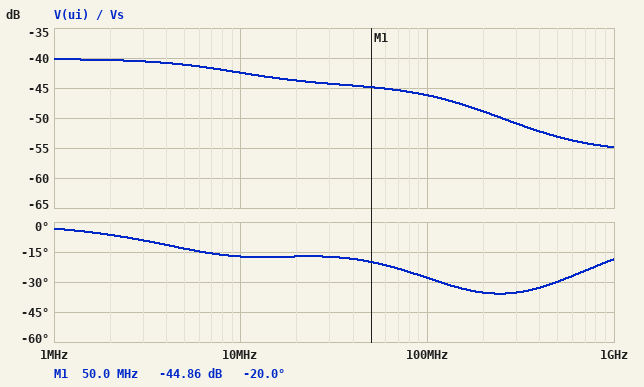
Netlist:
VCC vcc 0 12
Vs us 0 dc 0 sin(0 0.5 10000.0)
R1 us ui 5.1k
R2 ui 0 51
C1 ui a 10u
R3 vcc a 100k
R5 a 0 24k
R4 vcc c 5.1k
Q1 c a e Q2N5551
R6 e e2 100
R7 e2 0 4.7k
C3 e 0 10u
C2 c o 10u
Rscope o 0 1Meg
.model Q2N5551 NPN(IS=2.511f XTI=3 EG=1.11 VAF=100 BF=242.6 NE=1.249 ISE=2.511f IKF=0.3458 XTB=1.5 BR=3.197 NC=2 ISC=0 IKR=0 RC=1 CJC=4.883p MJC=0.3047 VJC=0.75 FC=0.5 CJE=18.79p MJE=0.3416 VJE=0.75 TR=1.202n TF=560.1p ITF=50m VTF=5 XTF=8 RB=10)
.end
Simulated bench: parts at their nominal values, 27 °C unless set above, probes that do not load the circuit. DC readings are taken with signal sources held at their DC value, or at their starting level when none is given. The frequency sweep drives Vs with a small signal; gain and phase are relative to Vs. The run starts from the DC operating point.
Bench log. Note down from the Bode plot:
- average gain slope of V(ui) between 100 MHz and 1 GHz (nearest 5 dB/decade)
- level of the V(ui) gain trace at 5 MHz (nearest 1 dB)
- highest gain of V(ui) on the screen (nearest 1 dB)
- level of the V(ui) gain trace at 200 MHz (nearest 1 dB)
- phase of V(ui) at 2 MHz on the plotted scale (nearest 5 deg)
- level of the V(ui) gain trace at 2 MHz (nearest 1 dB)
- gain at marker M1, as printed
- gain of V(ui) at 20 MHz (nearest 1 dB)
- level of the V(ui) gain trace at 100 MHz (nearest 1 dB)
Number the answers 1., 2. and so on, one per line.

1. -10 dB/decade
2. -41 dB
3. -40 dB
4. -49 dB
5. -5 deg
6. -40 dB
7. -44.86 dB
8. -44 dB
9. -46 dB
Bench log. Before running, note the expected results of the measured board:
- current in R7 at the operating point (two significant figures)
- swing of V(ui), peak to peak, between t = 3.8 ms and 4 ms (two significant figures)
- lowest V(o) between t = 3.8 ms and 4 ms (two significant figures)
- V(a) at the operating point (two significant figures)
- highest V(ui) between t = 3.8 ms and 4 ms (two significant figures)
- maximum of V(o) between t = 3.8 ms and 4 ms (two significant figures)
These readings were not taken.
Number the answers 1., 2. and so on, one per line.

1. 330 µA
2. 9.8 mV
3. -330 mV
4. 2.3 V
5. 4.9 mV
6. 300 mV
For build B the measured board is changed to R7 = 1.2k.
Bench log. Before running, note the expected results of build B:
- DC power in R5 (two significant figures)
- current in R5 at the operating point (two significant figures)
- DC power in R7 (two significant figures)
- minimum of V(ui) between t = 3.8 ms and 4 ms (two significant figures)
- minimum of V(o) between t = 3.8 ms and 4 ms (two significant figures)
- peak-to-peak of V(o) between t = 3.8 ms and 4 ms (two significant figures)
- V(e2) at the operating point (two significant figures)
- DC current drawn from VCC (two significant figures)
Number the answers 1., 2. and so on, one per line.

1. 190 µW
2. 89 µA
3. 1.5 mW
4. -4.9 mV
5. -1.0 V
6. 2.0 V
7. 1.3 V
8. 1.2 mA
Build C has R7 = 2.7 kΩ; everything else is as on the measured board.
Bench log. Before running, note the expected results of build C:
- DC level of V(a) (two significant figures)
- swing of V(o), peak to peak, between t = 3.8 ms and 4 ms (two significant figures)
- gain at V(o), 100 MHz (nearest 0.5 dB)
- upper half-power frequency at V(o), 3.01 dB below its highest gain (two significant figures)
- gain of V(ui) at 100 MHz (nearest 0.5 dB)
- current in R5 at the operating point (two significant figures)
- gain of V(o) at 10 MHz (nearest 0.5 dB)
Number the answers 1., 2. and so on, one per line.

1. 2.2 V
2. 1.0 V
3. -26.5 dB
4. 5.6 MHz
5. -47.5 dB
6. 93 µA
7. -6.0 dB
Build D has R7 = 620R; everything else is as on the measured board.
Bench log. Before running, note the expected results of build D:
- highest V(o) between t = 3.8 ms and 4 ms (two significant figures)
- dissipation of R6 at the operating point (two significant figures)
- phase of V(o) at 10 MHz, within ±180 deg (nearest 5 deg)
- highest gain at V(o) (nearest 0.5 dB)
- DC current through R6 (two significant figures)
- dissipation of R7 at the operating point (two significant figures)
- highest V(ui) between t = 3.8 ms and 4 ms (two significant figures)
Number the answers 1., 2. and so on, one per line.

1. 1.5 V
2. 340 µW
3. 95 deg
4. 10.0 dB
5. 1.8 mA
6. 2.1 mW
7. 4.4 mV
